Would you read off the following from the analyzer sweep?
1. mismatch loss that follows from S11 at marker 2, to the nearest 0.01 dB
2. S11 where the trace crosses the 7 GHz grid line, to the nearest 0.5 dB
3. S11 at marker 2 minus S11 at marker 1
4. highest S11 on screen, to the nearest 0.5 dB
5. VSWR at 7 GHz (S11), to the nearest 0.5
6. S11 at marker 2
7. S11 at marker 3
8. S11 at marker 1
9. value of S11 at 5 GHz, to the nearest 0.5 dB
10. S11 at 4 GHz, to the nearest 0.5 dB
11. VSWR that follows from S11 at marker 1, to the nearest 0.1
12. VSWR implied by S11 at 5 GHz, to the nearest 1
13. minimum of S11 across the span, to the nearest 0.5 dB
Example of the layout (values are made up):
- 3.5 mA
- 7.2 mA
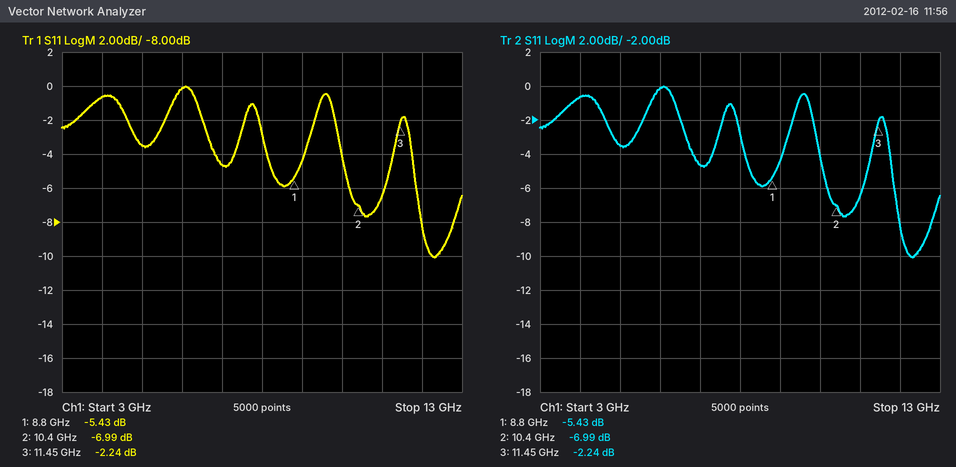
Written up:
- 0.97 dB
- -4.5 dB
- -1.56 dB
- 0.0 dB
- 4.0
- -6.99 dB
- -2.24 dB
- -5.43 dB
- -3.5 dB
- -0.5 dB
- 3.3
- 5
- -10.0 dB
